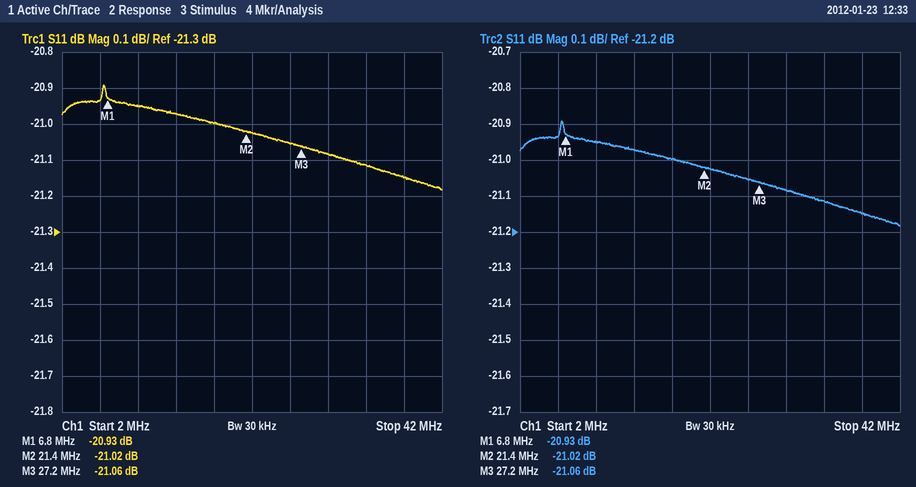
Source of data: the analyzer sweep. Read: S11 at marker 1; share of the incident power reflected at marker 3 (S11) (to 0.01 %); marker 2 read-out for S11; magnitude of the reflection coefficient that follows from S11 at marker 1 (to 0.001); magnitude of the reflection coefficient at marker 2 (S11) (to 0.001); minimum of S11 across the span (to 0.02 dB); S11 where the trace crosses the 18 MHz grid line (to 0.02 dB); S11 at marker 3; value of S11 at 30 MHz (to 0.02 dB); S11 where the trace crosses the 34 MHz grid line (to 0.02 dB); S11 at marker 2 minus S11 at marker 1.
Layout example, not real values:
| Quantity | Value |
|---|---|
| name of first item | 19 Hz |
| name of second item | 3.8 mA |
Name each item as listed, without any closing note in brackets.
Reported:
| Quantity | Value |
|---|---|
| S11 at marker 1 | -20.93 dB |
| share of the incident power reflected at marker 3 (S11) | 0.78 % |
| marker 2 read-out for S11 | -21.02 dB |
| magnitude of the reflection coefficient that follows from S11 at marker 1 | 0.090 |
| magnitude of the reflection coefficient at marker 2 (S11) | 0.089 |
| minimum of S11 across the span | -21.18 dB |
| S11 where the trace crosses the 18 MHz grid line | -21.00 dB |
| S11 at marker 3 | -21.06 dB |
| value of S11 at 30 MHz | -21.08 dB |
| S11 where the trace crosses the 34 MHz grid line | -21.12 dB |
| S11 at marker 2 minus S11 at marker 1 | -0.09 dB |
